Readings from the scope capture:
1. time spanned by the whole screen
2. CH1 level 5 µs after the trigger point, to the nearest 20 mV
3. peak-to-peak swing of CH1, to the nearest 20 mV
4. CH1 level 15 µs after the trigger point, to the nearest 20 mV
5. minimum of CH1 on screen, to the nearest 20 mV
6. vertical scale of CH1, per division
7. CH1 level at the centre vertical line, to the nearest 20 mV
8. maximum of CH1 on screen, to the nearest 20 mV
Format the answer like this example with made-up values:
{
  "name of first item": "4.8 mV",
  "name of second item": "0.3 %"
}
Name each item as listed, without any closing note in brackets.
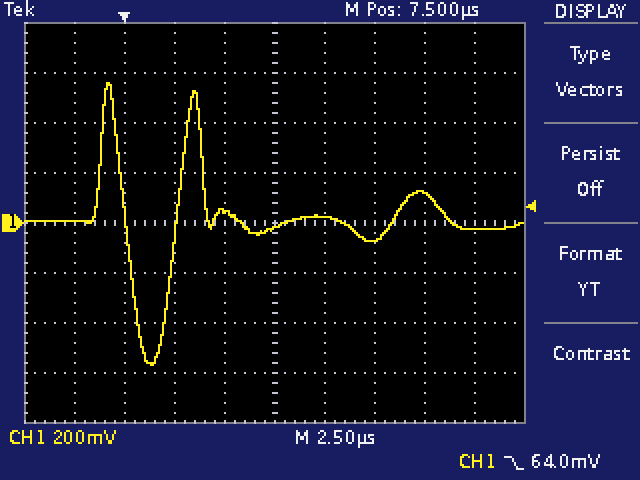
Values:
{
  "time spanned by the whole screen": "25 µs",
  "CH1 level 5 µs after the trigger point, to the nearest 20 mV": "40 mV",
  "peak-to-peak swing of CH1, to the nearest 20 mV": "1.12 V",
  "CH1 level 15 µs after the trigger point, to the nearest 20 mV": "120 mV",
  "minimum of CH1 on screen, to the nearest 20 mV": "-560 mV",
  "vertical scale of CH1, per division": "200 mV",
  "CH1 level at the centre vertical line, to the nearest 20 mV": "-20 mV",
  "maximum of CH1 on screen, to the nearest 20 mV": "560 mV"
}
